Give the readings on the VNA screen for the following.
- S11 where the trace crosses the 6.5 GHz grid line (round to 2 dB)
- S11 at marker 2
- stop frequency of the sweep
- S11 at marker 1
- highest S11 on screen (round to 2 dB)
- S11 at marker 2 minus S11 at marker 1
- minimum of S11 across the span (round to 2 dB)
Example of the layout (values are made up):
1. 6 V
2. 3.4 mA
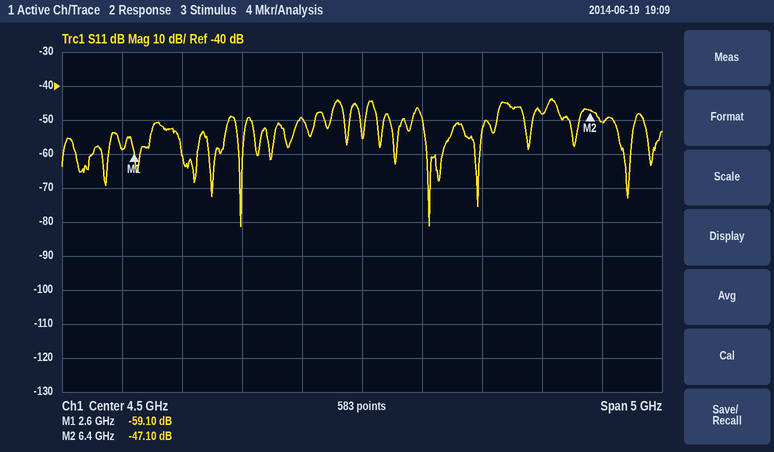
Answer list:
1. -50 dB
2. -47.10 dB
3. 7 GHz
4. -59.10 dB
5. -44 dB
6. 12.00 dB
7. -82 dB
